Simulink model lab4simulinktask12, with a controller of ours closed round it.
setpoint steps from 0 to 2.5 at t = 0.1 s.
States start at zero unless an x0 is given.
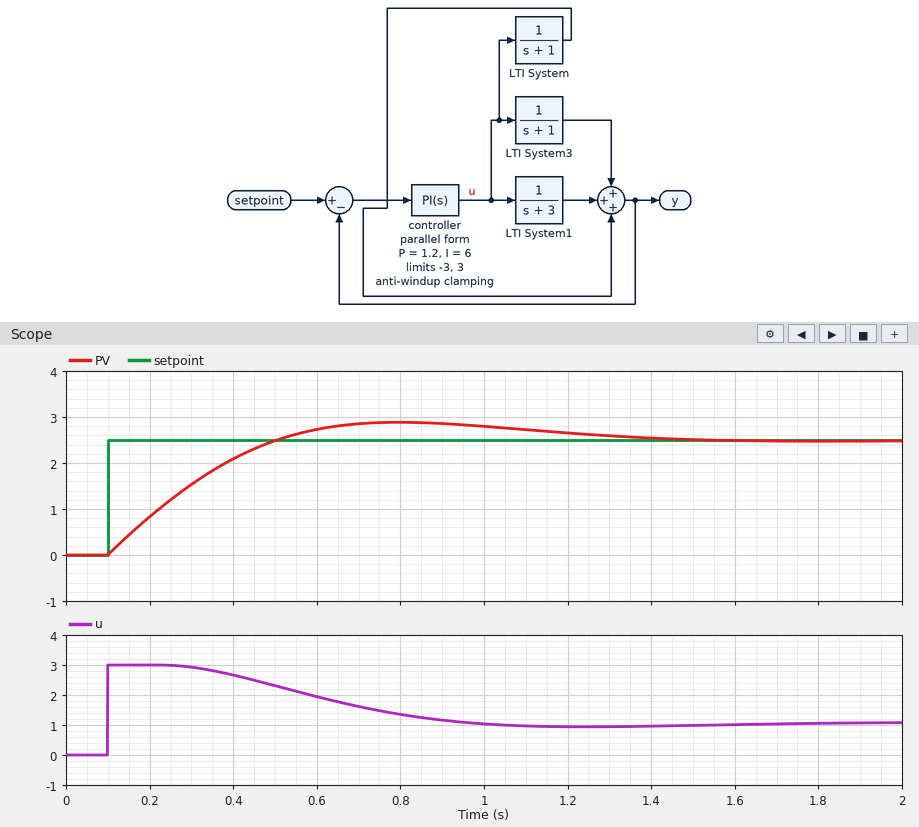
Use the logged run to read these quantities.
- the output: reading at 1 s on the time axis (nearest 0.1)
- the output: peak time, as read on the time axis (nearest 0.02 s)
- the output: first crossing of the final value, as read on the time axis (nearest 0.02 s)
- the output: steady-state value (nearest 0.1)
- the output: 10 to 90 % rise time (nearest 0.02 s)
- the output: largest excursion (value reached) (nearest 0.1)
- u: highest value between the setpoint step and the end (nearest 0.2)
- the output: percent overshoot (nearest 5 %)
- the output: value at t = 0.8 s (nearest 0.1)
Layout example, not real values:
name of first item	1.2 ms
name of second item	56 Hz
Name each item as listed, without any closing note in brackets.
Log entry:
the output: reading at 1 s on the time axis	2.8
the output: peak time, as read on the time axis	0.80 s
the output: first crossing of the final value, as read on the time axis	0.50 s
the output: steady-state value	2.5
the output: 10 to 90 % rise time	0.30 s
the output: largest excursion (value reached)	2.9
u: highest value between the setpoint step and the end	3.0
the output: percent overshoot	15 %
the output: value at t = 0.8 s	2.9
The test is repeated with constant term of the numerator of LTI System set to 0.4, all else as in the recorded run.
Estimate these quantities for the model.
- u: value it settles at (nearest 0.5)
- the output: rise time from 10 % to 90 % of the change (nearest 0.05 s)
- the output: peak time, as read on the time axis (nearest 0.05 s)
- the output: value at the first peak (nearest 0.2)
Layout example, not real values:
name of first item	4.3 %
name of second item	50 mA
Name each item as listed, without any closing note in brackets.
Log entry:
u: value it settles at	1.5
the output: rise time from 10 % to 90 % of the change	0.40 s
the output: peak time, as read on the time axis	1.00 s
the output: value at the first peak	2.8
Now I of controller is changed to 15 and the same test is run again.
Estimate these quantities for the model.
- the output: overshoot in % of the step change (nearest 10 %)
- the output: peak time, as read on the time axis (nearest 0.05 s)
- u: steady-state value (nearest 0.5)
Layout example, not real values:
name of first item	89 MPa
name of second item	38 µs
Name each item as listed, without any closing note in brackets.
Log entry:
the output: overshoot in % of the step change	20 %
the output: peak time, as read on the time axis	0.65 s
u: steady-state value	1.0
